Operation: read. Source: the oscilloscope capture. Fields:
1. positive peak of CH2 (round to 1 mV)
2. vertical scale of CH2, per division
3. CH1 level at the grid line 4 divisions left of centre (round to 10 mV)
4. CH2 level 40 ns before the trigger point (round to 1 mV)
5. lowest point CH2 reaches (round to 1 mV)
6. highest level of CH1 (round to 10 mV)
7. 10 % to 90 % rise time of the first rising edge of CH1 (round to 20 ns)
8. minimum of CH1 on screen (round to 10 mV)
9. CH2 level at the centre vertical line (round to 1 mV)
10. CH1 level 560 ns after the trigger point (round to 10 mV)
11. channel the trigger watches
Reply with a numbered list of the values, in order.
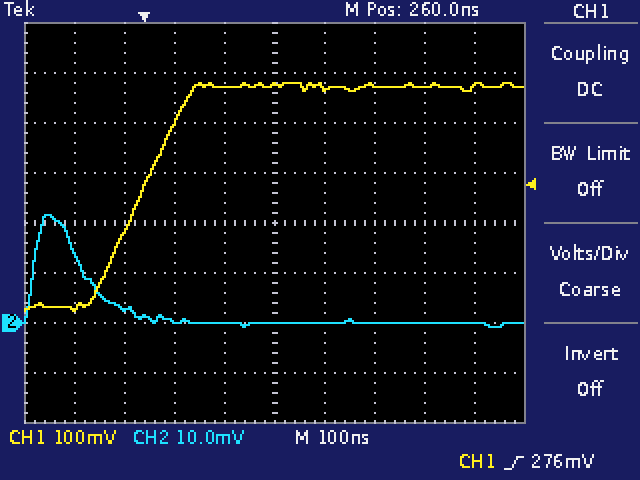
1. 22 mV
2. 10 mV
3. 30 mV
4. 3 mV
5. -1 mV
6. 480 mV
7. 160 ns
8. 20 mV
9. 0 mV
10. 470 mV
11. CH1
